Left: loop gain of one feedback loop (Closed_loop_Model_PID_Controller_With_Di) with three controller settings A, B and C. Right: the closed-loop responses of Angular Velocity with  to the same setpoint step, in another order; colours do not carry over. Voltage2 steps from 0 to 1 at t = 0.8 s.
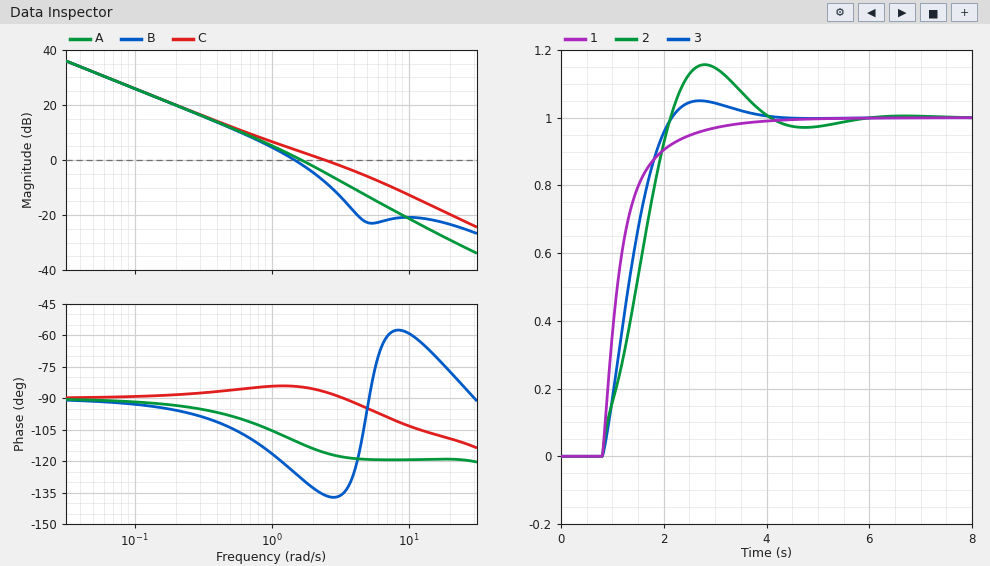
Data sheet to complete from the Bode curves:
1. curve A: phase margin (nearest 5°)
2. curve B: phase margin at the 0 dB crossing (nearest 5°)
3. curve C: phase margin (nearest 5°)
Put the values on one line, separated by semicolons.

70°; 55°; 95°
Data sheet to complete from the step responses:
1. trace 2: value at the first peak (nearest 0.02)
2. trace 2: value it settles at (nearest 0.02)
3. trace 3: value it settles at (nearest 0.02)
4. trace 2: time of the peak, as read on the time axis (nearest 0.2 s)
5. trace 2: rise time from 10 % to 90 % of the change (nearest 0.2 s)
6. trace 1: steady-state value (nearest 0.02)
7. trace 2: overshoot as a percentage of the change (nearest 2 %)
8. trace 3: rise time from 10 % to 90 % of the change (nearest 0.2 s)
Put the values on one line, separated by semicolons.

1.16; 1.00; 1.00; 2.8 s; 1.0 s; 1.00; 16 %; 1.0 s
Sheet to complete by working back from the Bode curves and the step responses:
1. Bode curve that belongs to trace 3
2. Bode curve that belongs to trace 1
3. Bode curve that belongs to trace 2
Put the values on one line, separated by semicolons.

A; C; B
